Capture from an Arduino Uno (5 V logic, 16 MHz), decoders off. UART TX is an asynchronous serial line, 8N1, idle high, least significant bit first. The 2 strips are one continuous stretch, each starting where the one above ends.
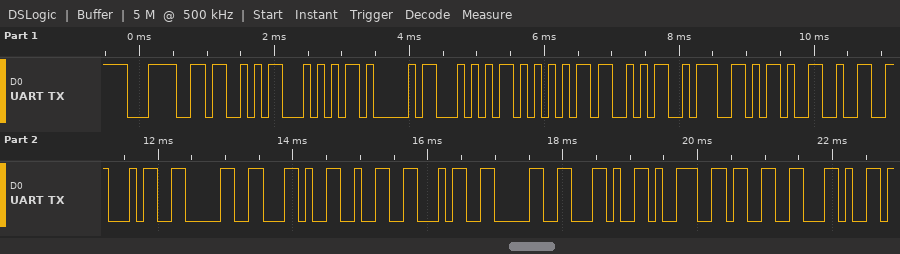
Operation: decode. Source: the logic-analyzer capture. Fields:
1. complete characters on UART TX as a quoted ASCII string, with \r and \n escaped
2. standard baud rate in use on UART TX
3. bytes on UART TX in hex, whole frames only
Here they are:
"<STATUS:-240,240,93,"
9600 baud
3C 53 54 41 54 55 53 3A 2D 32 34 30 2C 32 34 30 2C 39 33 2C
